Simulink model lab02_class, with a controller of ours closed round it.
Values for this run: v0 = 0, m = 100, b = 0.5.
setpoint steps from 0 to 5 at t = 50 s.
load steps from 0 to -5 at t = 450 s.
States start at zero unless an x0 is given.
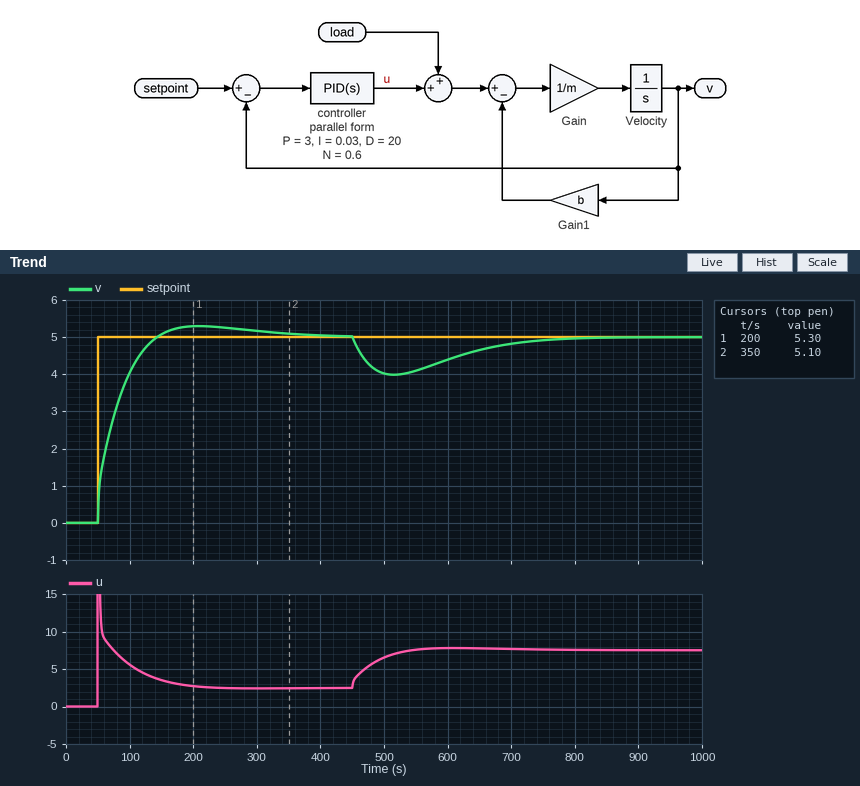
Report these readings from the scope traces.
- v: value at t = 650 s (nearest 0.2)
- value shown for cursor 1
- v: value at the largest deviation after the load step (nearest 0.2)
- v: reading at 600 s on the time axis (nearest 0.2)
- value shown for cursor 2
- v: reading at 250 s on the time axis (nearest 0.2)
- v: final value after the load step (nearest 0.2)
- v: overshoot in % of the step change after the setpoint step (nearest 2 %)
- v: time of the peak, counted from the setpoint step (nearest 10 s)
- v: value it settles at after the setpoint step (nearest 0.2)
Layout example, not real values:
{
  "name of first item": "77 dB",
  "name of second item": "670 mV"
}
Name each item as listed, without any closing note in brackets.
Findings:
{
  "v: value at t = 650 s": "4.6",
  "value shown for cursor 1": "5.30",
  "v: value at the largest deviation after the load step": "4.0",
  "v: reading at 600 s on the time axis": "4.4",
  "value shown for cursor 2": "5.10",
  "v: reading at 250 s on the time axis": "5.2",
  "v: final value after the load step": "5.0",
  "v: overshoot in % of the step change after the setpoint step": "6 %",
  "v: time of the peak, counted from the setpoint step": "160 s",
  "v: value it settles at after the setpoint step": "5.0"
}
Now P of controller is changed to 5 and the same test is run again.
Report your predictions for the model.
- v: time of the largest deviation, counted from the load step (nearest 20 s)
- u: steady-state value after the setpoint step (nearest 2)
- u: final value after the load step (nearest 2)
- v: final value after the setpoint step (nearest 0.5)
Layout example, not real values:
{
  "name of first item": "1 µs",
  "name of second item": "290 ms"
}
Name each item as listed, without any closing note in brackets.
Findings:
{
  "v: time of the largest deviation, counted from the load step": "60 s",
  "u: steady-state value after the setpoint step": "2",
  "u: final value after the load step": "8",
  "v: final value after the setpoint step": "5.0"
}
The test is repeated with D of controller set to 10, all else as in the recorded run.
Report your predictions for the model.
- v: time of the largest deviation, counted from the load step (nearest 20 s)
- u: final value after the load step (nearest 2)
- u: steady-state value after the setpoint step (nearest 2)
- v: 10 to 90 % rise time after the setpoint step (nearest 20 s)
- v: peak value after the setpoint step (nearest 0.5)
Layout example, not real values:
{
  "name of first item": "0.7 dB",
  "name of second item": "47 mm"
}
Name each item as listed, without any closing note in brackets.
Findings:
{
  "v: time of the largest deviation, counted from the load step": "60 s",
  "u: final value after the load step": "8",
  "u: steady-state value after the setpoint step": "2",
  "v: 10 to 90 % rise time after the setpoint step": "60 s",
  "v: peak value after the setpoint step": "5.5"
}
